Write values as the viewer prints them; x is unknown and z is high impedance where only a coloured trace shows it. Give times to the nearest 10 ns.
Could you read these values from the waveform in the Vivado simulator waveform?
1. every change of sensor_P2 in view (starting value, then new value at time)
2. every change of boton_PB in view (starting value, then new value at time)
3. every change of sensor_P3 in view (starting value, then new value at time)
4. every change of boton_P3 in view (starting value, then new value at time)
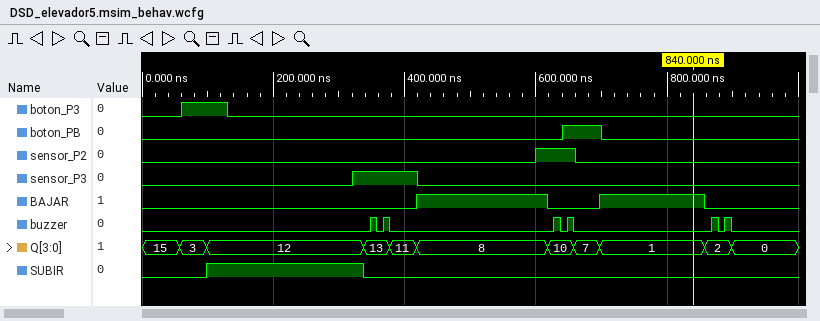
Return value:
0, 1 at 600 ns, 0 at 660 ns
0, 1 at 640 ns, 0 at 700 ns
0, 1 at 320 ns, 0 at 420 ns
0, 1 at 60 ns, 0 at 130 ns
